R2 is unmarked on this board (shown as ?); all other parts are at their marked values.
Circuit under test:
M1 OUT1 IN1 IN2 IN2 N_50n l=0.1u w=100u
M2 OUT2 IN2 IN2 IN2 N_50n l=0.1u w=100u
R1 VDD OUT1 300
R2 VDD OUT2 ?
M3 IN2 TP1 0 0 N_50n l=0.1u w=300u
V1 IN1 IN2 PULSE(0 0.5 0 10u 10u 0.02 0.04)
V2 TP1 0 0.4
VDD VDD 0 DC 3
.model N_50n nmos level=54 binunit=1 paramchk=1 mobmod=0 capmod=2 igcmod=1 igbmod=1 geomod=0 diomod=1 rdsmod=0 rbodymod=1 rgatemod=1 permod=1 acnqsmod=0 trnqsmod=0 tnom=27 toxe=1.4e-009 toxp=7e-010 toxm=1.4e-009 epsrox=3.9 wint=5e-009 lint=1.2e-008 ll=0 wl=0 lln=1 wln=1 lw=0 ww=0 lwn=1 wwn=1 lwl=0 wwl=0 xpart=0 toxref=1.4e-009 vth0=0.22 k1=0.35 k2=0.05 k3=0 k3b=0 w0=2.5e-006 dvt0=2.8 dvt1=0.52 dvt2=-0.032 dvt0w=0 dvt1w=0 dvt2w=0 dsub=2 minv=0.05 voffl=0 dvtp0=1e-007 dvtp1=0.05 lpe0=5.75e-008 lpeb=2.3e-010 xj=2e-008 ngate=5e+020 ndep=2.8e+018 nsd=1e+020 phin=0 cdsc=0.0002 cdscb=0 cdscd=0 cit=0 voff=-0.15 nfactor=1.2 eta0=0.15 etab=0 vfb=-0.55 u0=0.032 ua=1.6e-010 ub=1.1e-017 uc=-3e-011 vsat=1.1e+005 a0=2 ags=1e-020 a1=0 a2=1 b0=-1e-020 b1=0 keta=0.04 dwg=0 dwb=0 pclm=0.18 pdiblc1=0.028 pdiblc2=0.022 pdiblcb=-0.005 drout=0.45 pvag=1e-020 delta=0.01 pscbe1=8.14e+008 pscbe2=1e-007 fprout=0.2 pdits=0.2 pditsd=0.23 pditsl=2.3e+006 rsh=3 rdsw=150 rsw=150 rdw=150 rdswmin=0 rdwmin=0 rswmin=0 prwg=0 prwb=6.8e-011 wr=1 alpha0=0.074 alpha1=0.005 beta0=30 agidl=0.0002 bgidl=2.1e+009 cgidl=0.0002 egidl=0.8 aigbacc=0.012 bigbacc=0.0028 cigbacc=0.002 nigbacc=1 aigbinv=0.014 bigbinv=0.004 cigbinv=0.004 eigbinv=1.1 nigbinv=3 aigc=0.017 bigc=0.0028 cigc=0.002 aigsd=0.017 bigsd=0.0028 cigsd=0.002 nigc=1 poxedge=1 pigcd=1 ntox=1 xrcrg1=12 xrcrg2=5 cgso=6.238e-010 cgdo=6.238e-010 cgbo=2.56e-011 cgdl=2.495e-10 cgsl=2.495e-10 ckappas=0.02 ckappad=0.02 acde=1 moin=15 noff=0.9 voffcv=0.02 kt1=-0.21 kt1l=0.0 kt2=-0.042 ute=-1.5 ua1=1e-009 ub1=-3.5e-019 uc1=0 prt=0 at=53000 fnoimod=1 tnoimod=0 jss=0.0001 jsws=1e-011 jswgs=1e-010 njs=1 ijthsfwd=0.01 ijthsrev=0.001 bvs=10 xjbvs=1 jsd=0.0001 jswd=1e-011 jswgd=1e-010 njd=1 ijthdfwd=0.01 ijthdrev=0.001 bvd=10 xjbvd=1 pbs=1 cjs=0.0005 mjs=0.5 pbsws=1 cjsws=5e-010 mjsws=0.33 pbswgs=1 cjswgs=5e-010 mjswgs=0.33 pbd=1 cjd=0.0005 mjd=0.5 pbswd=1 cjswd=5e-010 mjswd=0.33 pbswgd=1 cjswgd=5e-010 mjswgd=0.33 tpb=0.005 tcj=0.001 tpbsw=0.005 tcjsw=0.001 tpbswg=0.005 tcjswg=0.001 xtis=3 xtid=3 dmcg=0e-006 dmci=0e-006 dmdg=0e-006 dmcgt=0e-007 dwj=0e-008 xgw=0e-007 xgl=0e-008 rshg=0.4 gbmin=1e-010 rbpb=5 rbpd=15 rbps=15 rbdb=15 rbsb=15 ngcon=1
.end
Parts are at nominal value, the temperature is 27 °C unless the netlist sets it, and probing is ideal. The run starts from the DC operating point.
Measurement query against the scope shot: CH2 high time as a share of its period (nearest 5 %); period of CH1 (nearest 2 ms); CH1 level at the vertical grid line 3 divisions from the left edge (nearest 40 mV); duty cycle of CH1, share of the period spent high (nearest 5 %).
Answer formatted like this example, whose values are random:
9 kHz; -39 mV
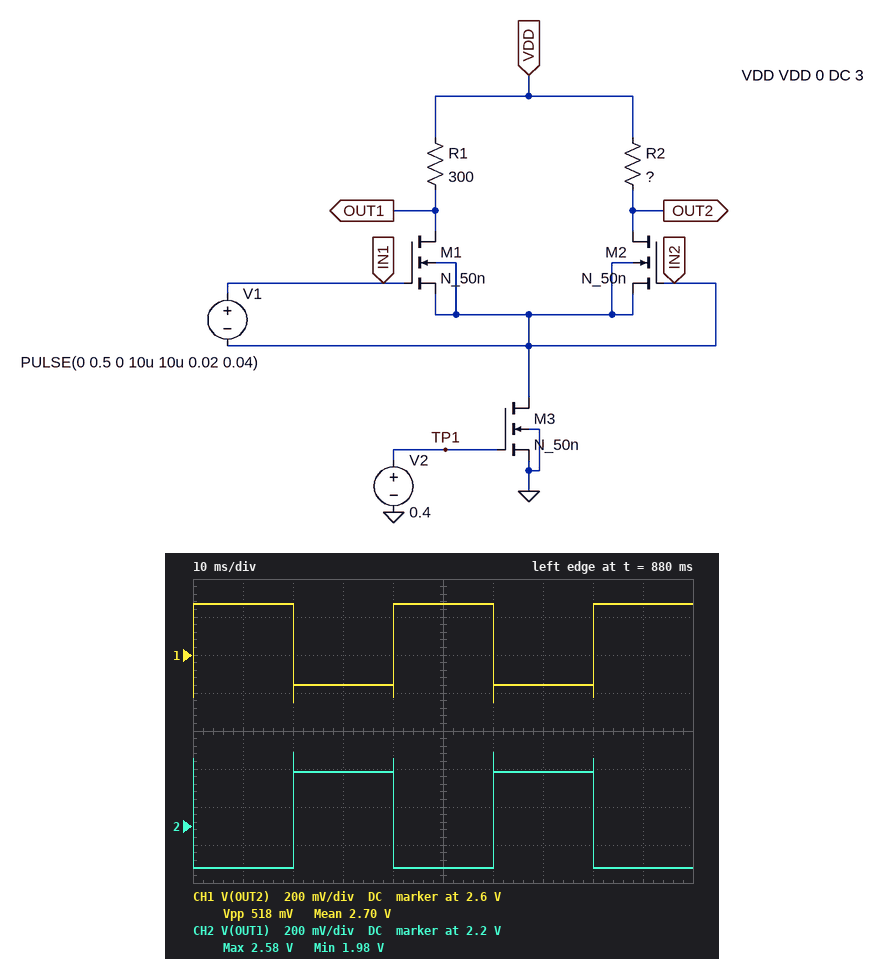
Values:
50 %; 40 ms; 2.44 V; 50 %
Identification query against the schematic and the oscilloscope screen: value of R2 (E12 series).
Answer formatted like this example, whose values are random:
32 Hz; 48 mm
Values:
470 Ω
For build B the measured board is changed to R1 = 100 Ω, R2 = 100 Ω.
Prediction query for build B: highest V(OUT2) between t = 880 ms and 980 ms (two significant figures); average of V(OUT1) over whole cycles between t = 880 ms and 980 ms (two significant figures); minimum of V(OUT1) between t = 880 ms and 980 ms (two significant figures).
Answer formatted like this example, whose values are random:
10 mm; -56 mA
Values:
3.0 V; 2.7 V; 2.6 V
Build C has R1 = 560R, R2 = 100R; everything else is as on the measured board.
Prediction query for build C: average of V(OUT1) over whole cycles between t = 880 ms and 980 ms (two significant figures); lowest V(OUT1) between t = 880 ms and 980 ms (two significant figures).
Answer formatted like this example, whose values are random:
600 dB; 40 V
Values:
2.0 V; 1.4 V
